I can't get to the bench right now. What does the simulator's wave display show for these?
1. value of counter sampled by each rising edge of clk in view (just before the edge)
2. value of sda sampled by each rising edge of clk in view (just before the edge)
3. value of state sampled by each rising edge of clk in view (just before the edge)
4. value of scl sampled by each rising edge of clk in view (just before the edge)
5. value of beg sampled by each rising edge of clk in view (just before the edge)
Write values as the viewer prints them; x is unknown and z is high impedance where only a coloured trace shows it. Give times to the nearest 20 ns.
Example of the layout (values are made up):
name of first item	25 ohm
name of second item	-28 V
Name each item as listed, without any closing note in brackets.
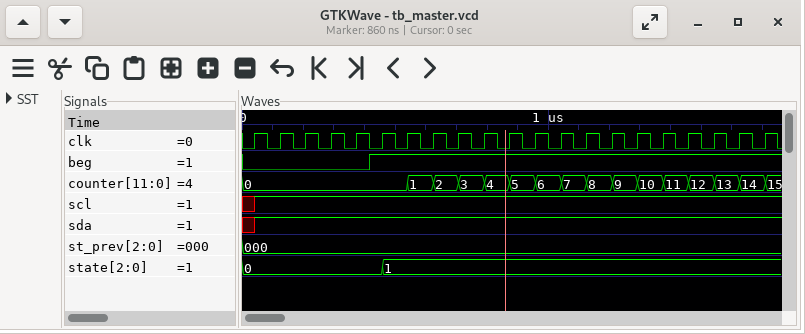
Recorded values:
value of counter sampled by each rising edge of clk in view	0, 0, 0, 0, 0, 0, 0, 1, 2, 3, 4, 5, 6, 7, 8, 9, 10, 11, 12, 13, 14
value of sda sampled by each rising edge of clk in view	x 1 1 1 1 1 1 1 1 1 1 1 1 1 1 1 1 1 1 1 1
value of state sampled by each rising edge of clk in view	0, 0, 0, 0, 0, 0, 1, 1, 1, 1, 1, 1, 1, 1, 1, 1, 1, 1, 1, 1, 1
value of scl sampled by each rising edge of clk in view	x 1 1 1 1 1 1 1 1 1 1 1 1 1 1 1 1 1 1 1 1
value of beg sampled by each rising edge of clk in view	0 0 0 0 0 1 1 1 1 1 1 1 1 1 1 1 1 1 1 1 1
